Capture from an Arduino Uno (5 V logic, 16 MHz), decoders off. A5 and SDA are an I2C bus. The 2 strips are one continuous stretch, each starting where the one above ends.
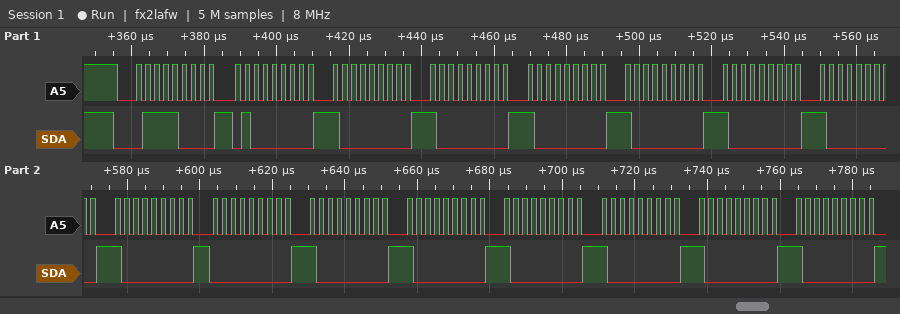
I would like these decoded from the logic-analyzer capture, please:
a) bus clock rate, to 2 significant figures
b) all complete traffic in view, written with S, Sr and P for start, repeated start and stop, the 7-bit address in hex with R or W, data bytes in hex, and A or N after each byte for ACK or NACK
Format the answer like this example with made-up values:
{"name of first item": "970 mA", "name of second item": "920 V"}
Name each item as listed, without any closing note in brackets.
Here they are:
{"bus clock rate, to 2 significant figures": "400 kHz", "all complete traffic in view, written with S, Sr and P for start, repeated start and stop, the 7-bit address in hex with R or W, data bytes in hex, and A or N after each byte for ACK or NACK": "S 3CW A 40 A 80 A 80 A 80 A 80 A 80 A 80 A 80 A 00 A 80 A 80 A 80 A 80 A 80 A 80 A"}
